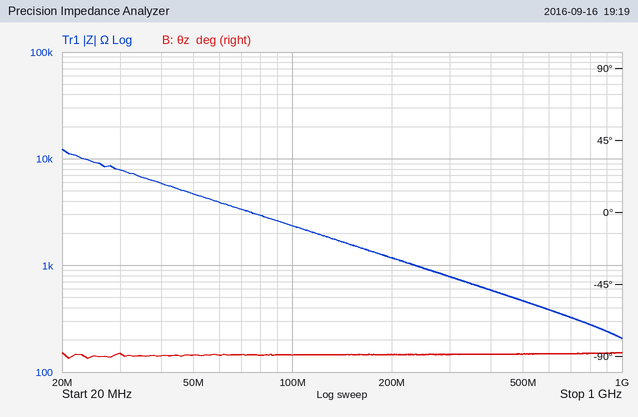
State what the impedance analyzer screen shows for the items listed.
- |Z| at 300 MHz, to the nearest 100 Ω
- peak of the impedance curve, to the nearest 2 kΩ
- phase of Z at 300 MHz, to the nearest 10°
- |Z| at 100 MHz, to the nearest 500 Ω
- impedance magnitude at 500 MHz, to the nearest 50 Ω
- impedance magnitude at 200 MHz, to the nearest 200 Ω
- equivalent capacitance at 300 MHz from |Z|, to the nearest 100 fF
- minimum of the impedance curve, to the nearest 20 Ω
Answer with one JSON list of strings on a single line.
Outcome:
["800 Ω", "12 kΩ", "-90°", "2.5 kΩ", "450 Ω", "1.2 kΩ", "700 fF", "200 Ω"]
